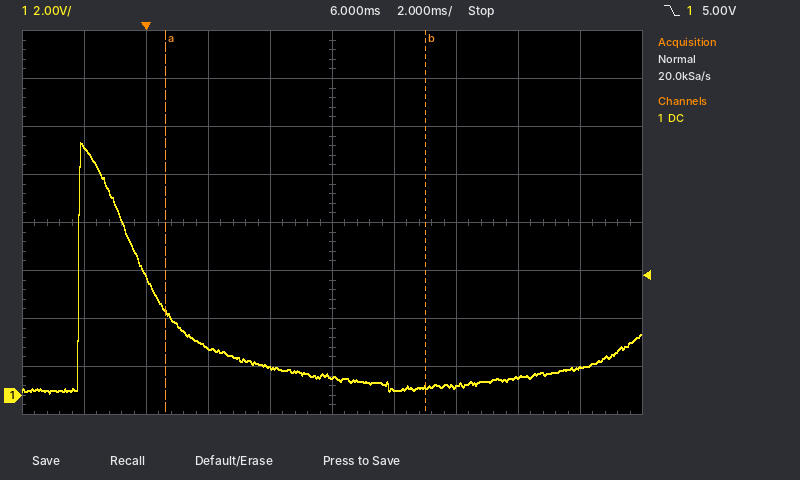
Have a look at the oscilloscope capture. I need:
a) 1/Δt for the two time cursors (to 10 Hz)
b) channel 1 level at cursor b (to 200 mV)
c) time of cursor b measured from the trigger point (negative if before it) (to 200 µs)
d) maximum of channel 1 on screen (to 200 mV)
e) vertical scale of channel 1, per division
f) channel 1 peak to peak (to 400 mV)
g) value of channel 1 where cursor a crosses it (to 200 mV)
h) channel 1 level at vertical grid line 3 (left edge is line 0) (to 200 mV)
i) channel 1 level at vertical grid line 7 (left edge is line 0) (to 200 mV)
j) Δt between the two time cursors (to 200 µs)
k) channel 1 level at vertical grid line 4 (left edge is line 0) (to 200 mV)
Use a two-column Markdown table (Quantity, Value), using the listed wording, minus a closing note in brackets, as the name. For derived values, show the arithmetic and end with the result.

| Quantity | Value |
|---|---|
| 1/Δt for the two time cursors | 1 / 8.4 ms ≈ 120 Hz |
| channel 1 level at cursor b | 400 mV |
| time of cursor b measured from the trigger point (negative if before it) | +9.0 ms |
| maximum of channel 1 on screen | 10.6 V |
| vertical scale of channel 1, per division | 2 V |
| channel 1 peak to peak | 10.4 V |
| value of channel 1 where cursor a crosses it | 3.6 V |
| channel 1 level at vertical grid line 3 (left edge is line 0) | 2.0 V |
| channel 1 level at vertical grid line 7 (left edge is line 0) | 400 mV |
| Δt between the two time cursors | 8.4 ms |
| channel 1 level at vertical grid line 4 (left edge is line 0) | 1.2 V |
